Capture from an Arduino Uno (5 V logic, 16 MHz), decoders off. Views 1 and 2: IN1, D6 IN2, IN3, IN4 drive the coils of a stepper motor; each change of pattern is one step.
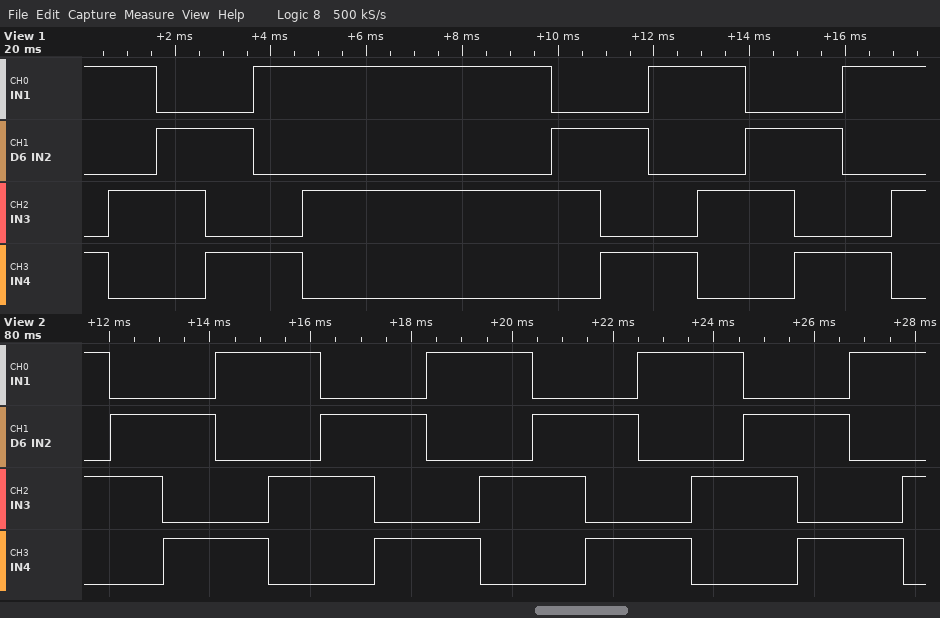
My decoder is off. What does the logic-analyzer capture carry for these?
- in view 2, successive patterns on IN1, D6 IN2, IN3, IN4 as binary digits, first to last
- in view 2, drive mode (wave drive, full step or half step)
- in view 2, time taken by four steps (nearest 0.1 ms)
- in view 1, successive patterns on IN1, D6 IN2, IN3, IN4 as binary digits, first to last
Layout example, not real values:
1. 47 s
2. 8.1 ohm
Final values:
1. 1010 0110 0101 1001 1010 0110 0101 1001 1010 0110 0101 1001 1010 0110 0101 1001 1010
2. full step
3. 4.2 ms
4. 1001 1010 0110 0101 1001 1010 0110 0101 1001 1010 0110 0101 1001 1010
